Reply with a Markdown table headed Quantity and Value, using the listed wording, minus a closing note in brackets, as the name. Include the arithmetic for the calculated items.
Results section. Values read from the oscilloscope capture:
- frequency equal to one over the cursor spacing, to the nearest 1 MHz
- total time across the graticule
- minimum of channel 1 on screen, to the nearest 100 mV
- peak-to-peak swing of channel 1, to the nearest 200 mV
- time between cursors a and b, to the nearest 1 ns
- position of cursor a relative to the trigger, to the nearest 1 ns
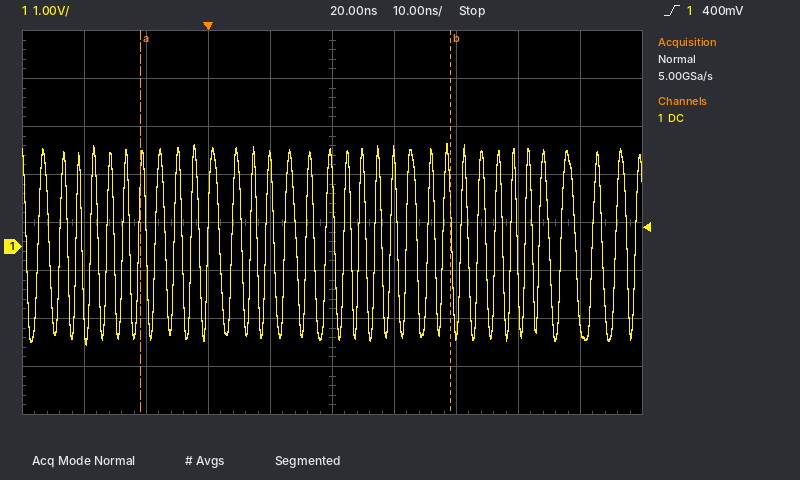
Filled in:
| Quantity | Value |
|---|---|
| frequency equal to one over the cursor spacing, to the nearest 1 MHz | 1 / 50 ns ≈ 20 MHz |
| total time across the graticule | 100 ns |
| minimum of channel 1 on screen, to the nearest 100 mV | -2.0 V |
| peak-to-peak swing of channel 1, to the nearest 200 mV | 4.2 V |
| time between cursors a and b, to the nearest 1 ns | 50 ns |
| position of cursor a relative to the trigger, to the nearest 1 ns | -11 ns |
